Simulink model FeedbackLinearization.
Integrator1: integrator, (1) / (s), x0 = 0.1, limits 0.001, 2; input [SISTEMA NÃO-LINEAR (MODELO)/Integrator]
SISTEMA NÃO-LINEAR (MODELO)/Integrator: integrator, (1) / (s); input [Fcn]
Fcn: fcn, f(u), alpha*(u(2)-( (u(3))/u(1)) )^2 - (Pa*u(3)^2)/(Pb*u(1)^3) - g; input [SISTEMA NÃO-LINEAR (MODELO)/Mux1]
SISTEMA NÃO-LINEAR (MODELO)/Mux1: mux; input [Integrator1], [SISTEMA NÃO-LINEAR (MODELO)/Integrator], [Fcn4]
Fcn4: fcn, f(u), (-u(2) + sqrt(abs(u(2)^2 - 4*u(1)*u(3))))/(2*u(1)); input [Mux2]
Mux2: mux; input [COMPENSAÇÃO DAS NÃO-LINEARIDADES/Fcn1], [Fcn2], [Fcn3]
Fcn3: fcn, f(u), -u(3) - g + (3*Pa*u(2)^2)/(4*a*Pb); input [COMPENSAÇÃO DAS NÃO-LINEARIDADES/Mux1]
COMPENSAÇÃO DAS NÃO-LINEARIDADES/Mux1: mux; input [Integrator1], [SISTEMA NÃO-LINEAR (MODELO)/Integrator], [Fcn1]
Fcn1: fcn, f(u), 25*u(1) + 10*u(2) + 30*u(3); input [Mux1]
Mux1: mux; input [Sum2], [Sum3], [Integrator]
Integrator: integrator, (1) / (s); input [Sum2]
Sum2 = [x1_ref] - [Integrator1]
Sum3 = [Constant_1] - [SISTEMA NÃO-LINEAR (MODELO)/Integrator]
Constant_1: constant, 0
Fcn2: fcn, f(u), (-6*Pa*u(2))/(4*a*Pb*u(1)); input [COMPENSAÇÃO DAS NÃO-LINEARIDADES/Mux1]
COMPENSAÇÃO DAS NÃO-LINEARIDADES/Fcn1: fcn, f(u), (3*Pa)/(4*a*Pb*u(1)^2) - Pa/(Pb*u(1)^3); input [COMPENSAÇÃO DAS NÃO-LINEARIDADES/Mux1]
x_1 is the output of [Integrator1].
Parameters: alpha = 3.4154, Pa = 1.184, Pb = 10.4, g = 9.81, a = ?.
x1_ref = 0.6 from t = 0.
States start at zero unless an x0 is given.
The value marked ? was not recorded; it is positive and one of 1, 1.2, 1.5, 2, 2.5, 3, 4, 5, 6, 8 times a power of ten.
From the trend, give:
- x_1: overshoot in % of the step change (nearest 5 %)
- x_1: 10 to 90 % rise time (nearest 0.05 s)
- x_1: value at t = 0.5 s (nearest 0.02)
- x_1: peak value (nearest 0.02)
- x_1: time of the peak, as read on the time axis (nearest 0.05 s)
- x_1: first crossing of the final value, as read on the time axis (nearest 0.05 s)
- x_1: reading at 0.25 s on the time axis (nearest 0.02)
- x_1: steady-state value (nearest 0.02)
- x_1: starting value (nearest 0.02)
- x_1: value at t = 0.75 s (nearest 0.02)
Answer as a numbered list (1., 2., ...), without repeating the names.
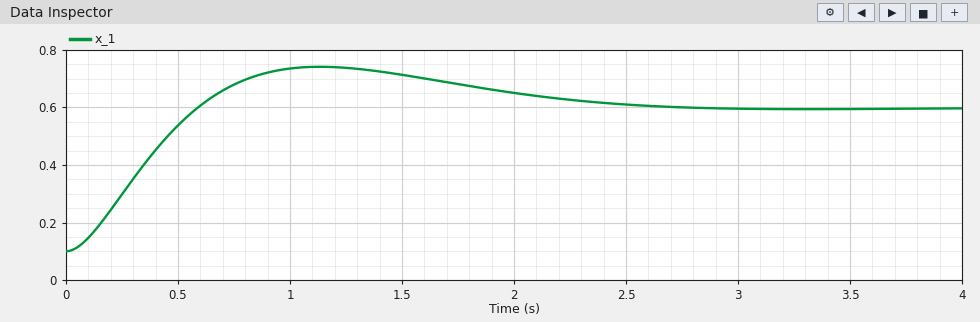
1. 30 %
2. 0.40 s
3. 0.54
4. 0.74
5. 1.15 s
6. 0.60 s
7. 0.30
8. 0.60
9. 0.10
10. 0.68
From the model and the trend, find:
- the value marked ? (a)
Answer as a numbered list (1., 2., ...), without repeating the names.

1. 0.025
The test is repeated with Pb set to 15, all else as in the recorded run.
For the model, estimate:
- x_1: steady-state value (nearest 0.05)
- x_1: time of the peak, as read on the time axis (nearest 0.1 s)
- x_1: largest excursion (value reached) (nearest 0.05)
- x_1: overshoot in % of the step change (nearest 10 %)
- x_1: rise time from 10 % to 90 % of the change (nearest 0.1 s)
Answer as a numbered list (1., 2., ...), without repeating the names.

1. 0.60
2. 1.0 s
3. 0.80
4. 40 %
5. 0.3 s
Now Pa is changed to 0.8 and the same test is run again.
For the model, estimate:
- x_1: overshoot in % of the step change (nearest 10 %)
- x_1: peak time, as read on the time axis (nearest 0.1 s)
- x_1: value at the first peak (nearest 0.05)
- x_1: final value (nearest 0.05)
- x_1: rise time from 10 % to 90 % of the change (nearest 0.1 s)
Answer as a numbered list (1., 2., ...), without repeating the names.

1. 40 %
2. 1.0 s
3. 0.80
4. 0.60
5. 0.3 s
